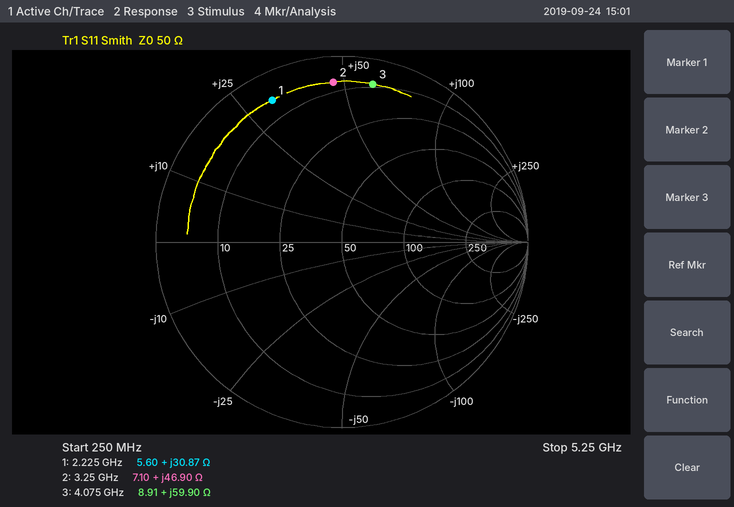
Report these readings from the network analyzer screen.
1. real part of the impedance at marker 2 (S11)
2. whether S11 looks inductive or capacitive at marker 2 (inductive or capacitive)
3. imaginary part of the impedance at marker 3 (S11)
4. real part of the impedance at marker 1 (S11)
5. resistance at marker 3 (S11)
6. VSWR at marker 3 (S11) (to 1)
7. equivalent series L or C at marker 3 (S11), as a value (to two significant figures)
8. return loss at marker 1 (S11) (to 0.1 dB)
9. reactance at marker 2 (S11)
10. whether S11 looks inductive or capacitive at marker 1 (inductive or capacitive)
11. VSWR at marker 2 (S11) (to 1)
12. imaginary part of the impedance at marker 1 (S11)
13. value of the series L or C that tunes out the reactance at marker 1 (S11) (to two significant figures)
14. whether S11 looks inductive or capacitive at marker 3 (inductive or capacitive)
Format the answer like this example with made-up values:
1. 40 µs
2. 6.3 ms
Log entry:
1. 7.10 Ω
2. inductive
3. +59.90 Ω
4. 5.60 Ω
5. 8.91 Ω
6. 14
7. 2.3 nH
8. 1.4 dB
9. +46.90 Ω
10. inductive
11. 13
12. +30.87 Ω
13. 2.3 pF
14. inductive
